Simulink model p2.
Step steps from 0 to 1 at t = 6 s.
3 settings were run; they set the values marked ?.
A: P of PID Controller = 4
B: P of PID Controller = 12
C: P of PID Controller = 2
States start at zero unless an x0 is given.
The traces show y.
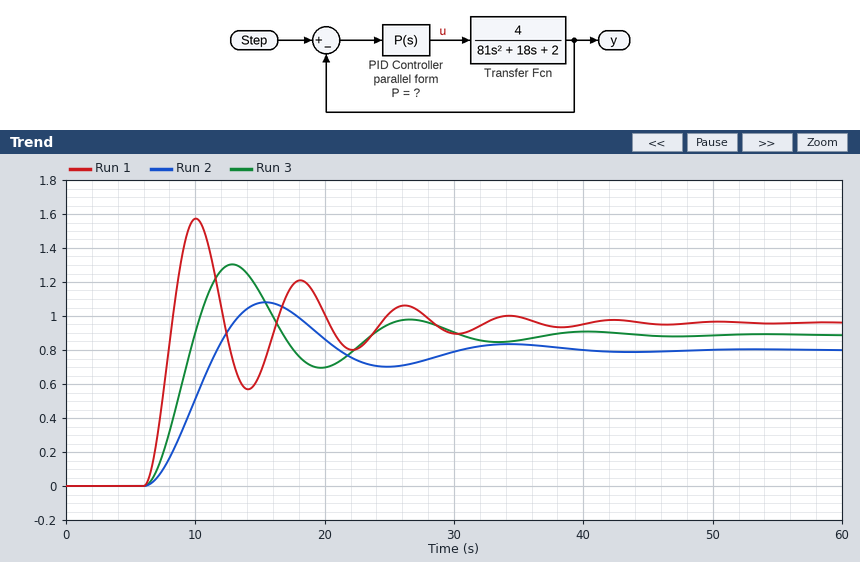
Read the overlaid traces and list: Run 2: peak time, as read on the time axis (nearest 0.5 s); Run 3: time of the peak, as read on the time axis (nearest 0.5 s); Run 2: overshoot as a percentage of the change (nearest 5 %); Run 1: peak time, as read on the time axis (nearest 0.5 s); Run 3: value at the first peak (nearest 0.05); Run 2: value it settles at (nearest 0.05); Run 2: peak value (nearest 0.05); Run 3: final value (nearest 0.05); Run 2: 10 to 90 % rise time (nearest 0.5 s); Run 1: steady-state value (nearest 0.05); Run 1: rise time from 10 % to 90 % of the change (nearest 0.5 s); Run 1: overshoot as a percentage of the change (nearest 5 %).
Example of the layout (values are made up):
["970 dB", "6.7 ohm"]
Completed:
["15.5 s", "13.0 s", "35 %", "10.0 s", "1.30", "0.80", "1.10", "0.90", "4.0 s", "0.95", "1.5 s", "65 %"]
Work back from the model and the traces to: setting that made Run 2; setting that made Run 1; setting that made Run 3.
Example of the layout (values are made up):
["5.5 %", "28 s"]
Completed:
["C", "B", "A"]
